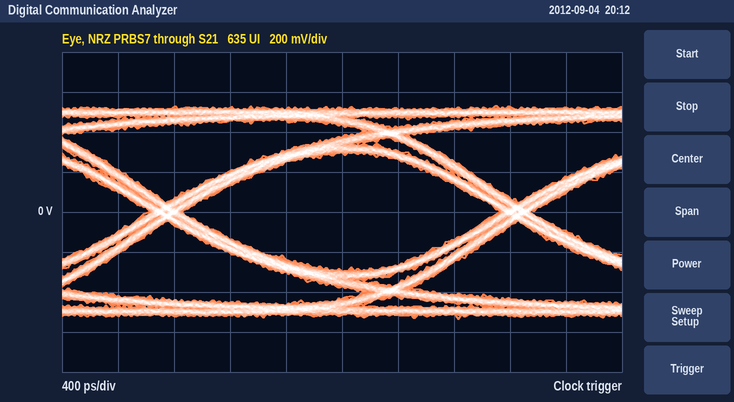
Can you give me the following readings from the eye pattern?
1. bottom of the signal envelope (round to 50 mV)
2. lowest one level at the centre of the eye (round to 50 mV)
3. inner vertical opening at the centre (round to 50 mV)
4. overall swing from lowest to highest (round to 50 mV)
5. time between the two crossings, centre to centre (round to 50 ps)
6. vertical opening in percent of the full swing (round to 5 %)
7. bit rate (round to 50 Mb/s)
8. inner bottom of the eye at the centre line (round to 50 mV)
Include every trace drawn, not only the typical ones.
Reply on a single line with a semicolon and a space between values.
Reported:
-550 mV; 300 mV; 600 mV; 1.05 V; 2.50 ns; 55 %; 400 Mb/s; -300 mV
